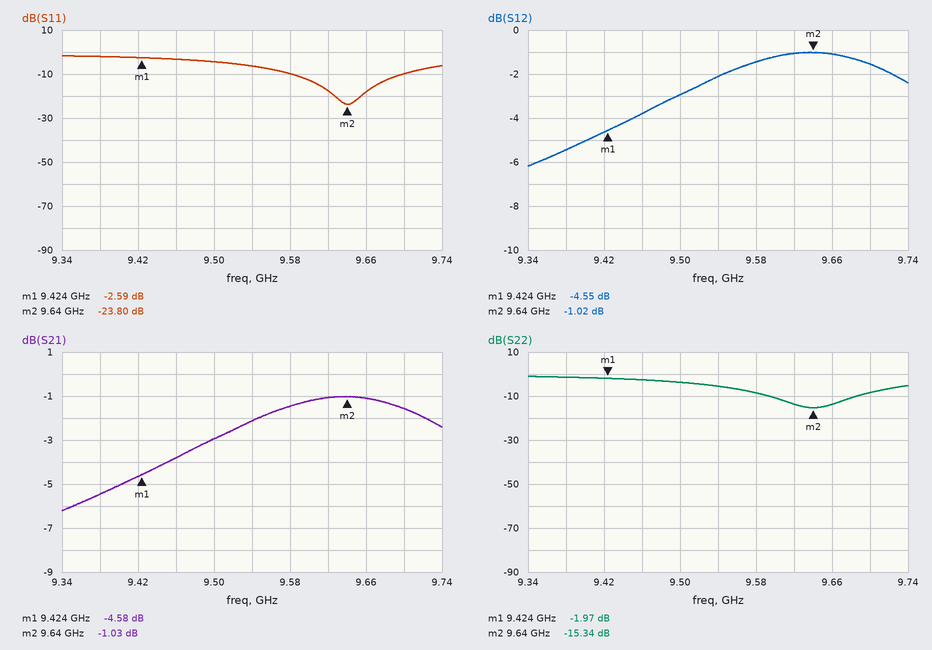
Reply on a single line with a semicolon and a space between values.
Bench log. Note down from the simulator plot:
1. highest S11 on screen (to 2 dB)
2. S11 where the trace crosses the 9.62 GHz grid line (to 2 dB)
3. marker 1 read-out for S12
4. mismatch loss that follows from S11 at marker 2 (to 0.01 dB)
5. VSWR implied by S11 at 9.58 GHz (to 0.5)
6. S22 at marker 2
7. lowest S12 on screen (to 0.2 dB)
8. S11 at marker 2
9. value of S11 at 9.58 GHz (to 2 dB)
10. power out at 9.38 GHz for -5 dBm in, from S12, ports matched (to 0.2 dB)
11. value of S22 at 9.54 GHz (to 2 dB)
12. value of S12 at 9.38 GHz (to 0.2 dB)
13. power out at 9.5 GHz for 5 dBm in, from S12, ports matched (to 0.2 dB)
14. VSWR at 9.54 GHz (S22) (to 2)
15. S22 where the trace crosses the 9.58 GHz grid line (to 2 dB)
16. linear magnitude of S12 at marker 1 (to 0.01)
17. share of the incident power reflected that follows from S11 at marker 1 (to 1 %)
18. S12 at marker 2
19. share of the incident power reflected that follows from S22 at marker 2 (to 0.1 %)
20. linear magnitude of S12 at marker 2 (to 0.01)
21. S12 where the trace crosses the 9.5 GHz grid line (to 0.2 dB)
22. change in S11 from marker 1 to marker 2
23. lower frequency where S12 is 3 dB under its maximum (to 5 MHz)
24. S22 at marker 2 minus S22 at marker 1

-2 dB; -18 dB; -4.55 dB; 0.02 dB; 2.0; -15.34 dB; -6.2 dB; -23.80 dB; -10 dB; -10.4 dBm; -6 dB; -5.4 dB; 2.0 dBm; 4; -8 dB; 0.59; 55 %; -1.02 dB; 2.9 %; 0.89; -3.0 dB; -21.21 dB; 9.450 GHz; -13.37 dB
